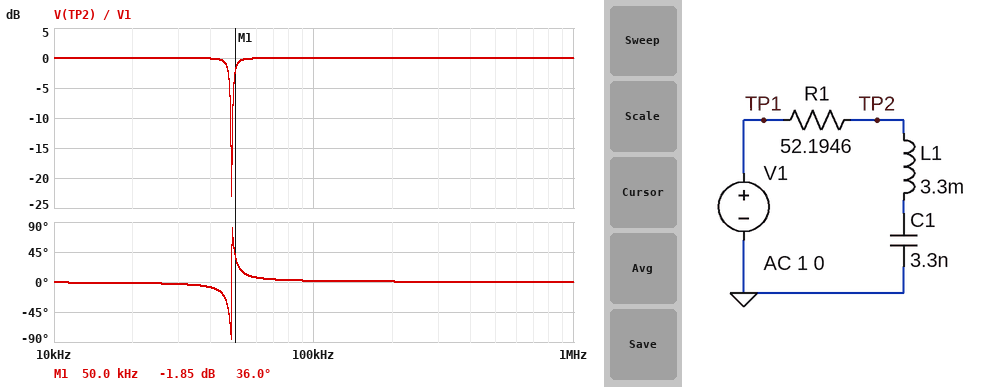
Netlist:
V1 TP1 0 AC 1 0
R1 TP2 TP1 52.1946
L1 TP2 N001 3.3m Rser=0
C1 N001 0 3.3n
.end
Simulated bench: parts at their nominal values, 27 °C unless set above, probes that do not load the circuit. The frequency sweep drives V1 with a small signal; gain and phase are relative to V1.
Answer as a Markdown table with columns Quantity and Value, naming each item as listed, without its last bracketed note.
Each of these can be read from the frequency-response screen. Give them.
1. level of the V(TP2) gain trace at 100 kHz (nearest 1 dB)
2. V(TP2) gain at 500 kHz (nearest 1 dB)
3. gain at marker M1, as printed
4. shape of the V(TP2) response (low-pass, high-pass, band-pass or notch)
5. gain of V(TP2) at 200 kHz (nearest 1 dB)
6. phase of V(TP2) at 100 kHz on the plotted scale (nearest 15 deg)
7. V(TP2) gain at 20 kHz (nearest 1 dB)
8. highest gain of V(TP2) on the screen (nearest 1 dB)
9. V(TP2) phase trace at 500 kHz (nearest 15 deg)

| Quantity | Value |
|---|---|
| level of the V(TP2) gain trace at 100 kHz | 0 dB |
| V(TP2) gain at 500 kHz | 0 dB |
| gain at marker M1, as printed | -1.85 dB |
| shape of the V(TP2) response | notch |
| gain of V(TP2) at 200 kHz | 0 dB |
| phase of V(TP2) at 100 kHz on the plotted scale | 0 deg |
| V(TP2) gain at 20 kHz | 0 dB |
| highest gain of V(TP2) on the screen | 0 dB |
| V(TP2) phase trace at 500 kHz | 0 deg |
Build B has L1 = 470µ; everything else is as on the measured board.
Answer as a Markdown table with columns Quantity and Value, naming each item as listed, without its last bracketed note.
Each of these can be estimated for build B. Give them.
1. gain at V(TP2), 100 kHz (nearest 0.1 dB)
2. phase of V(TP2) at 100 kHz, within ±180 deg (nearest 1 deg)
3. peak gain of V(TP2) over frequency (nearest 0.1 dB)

| Quantity | Value |
|---|---|
| gain at V(TP2), 100 kHz | -0.3 dB |
| phase of V(TP2) at 100 kHz, within ±180 deg | -16 deg |
| peak gain of V(TP2) over frequency | 0 dB |
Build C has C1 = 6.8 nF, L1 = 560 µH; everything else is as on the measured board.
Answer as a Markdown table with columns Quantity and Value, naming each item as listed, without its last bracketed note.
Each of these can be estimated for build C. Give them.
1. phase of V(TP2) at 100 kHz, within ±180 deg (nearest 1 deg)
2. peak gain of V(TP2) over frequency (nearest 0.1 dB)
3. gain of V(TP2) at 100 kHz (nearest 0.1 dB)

| Quantity | Value |
|---|---|
| phase of V(TP2) at 100 kHz, within ±180 deg | 24 deg |
| peak gain of V(TP2) over frequency | 0 dB |
| gain of V(TP2) at 100 kHz | -0.8 dB |
